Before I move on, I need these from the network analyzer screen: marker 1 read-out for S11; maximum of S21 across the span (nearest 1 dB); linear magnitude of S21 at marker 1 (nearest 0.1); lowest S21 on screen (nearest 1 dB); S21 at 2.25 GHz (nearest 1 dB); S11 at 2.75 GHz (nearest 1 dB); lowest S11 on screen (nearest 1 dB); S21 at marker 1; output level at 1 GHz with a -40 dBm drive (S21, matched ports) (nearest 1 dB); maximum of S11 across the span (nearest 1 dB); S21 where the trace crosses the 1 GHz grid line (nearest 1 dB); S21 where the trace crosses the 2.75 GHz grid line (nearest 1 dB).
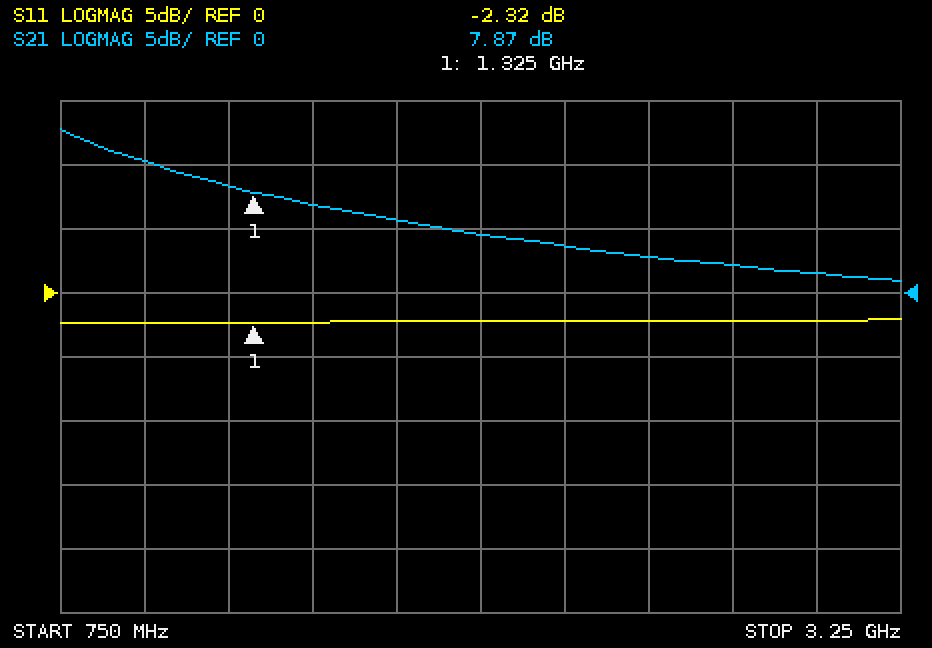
-2.32 dB
13 dB
2.5
1 dB
4 dB
-2 dB
-2 dB
7.87 dB
-30 dBm
-2 dB
10 dB
2 dB
